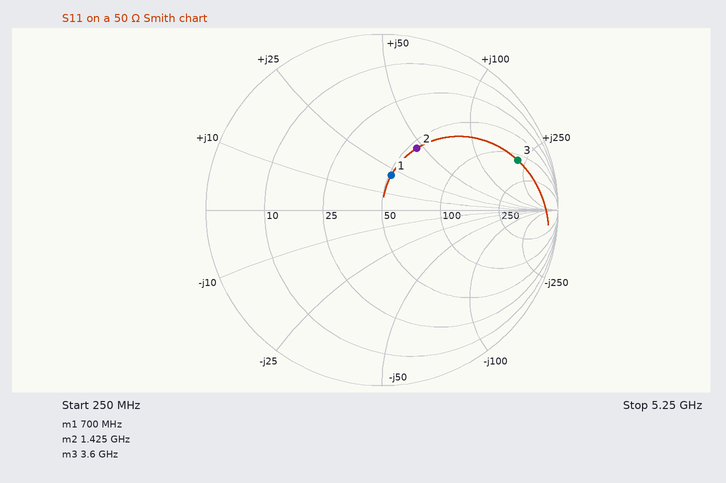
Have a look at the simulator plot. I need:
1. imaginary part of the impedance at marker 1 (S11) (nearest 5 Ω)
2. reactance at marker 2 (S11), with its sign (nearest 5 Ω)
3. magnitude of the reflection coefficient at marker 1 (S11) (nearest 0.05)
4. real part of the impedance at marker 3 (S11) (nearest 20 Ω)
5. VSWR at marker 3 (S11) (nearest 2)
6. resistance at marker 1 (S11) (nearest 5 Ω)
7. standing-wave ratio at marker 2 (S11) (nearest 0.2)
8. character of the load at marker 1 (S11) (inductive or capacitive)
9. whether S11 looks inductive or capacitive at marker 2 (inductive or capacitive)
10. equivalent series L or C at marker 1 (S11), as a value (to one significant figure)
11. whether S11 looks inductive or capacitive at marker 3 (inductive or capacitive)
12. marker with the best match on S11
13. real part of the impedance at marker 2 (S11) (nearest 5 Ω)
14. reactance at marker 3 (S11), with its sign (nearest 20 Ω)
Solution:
+20 Ω
+45 Ω
0.20
120 Ω
10
50 Ω
2.4
inductive
inductive
5 nH
inductive
marker 1
55 Ω
+220 Ω
